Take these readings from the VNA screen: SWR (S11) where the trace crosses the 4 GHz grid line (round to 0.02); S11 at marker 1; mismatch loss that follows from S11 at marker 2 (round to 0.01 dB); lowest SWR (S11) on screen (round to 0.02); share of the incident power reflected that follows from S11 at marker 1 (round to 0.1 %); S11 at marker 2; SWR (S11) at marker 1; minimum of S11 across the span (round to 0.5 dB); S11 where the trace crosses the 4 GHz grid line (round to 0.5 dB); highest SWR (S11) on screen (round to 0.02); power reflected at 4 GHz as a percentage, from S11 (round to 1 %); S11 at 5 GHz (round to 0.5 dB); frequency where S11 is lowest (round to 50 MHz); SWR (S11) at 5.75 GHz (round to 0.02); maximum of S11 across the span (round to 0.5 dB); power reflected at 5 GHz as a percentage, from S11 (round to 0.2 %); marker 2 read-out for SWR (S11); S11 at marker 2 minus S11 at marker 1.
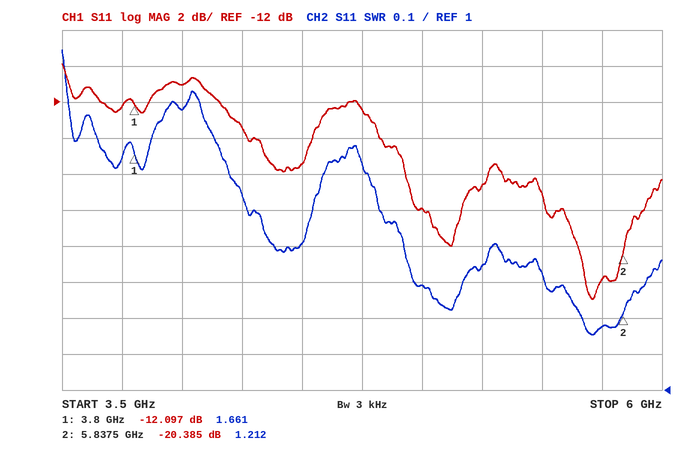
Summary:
1.78
-12.097 dB
0.04 dB
1.16
6.2 %
-20.385 dB
1.661
-23.0 dB
-11.0 dB
1.94
8 %
-18.0 dB
5.70 GHz
1.18
-10.0 dB
1.6 %
1.212
-8.288 dB
